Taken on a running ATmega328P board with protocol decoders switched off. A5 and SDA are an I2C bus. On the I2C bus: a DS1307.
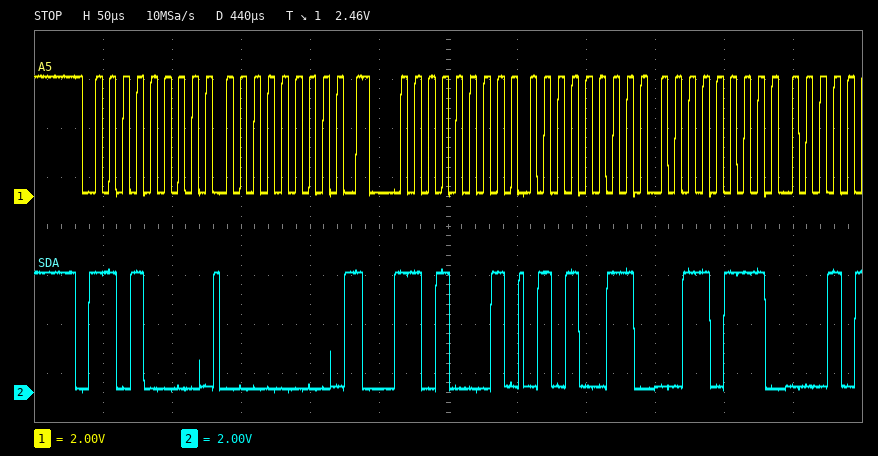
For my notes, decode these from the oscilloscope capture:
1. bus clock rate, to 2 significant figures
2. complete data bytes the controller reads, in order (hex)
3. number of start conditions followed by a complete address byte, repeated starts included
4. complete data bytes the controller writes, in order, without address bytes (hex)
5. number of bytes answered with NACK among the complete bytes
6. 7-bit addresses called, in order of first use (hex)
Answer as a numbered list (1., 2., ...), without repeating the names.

1. 100 kHz
2. 53 37
3. 2
4. 00
5. 0
6. 0x68
